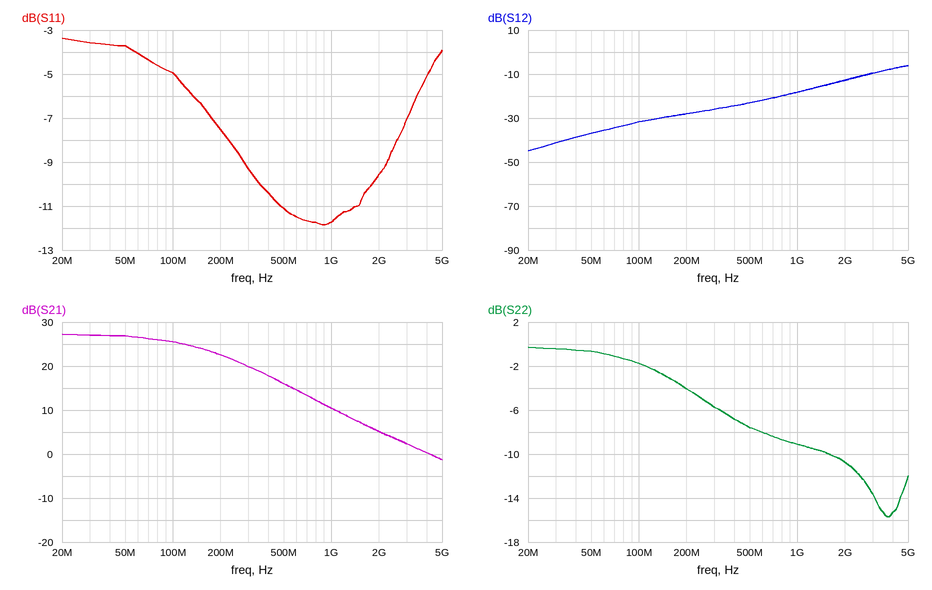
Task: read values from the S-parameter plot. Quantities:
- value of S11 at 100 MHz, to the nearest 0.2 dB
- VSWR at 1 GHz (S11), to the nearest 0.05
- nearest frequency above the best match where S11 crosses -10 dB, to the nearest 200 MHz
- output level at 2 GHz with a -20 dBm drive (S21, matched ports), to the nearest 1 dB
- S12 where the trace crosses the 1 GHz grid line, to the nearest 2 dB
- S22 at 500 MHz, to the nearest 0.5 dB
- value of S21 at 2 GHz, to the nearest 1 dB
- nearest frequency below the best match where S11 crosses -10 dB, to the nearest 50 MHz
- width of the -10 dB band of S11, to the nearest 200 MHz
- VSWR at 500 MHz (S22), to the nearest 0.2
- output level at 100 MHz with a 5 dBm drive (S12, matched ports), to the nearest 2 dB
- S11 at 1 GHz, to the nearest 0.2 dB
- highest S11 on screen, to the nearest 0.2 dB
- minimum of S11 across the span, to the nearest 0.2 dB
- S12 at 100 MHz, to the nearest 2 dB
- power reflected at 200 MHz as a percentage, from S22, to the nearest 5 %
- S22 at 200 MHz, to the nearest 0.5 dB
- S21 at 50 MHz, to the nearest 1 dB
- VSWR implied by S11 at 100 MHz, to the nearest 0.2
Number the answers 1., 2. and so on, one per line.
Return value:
1. -5.0 dB
2. 1.70
3. 1.8 GHz
4. -15 dBm
5. -18 dB
6. -7.5 dB
7. 5 dB
8. 350 MHz
9. 1.4 GHz
10. 2.4
11. -26 dBm
12. -11.8 dB
13. -3.4 dB
14. -11.8 dB
15. -32 dB
16. 40 %
17. -4.0 dB
18. 27 dB
19. 3.6
